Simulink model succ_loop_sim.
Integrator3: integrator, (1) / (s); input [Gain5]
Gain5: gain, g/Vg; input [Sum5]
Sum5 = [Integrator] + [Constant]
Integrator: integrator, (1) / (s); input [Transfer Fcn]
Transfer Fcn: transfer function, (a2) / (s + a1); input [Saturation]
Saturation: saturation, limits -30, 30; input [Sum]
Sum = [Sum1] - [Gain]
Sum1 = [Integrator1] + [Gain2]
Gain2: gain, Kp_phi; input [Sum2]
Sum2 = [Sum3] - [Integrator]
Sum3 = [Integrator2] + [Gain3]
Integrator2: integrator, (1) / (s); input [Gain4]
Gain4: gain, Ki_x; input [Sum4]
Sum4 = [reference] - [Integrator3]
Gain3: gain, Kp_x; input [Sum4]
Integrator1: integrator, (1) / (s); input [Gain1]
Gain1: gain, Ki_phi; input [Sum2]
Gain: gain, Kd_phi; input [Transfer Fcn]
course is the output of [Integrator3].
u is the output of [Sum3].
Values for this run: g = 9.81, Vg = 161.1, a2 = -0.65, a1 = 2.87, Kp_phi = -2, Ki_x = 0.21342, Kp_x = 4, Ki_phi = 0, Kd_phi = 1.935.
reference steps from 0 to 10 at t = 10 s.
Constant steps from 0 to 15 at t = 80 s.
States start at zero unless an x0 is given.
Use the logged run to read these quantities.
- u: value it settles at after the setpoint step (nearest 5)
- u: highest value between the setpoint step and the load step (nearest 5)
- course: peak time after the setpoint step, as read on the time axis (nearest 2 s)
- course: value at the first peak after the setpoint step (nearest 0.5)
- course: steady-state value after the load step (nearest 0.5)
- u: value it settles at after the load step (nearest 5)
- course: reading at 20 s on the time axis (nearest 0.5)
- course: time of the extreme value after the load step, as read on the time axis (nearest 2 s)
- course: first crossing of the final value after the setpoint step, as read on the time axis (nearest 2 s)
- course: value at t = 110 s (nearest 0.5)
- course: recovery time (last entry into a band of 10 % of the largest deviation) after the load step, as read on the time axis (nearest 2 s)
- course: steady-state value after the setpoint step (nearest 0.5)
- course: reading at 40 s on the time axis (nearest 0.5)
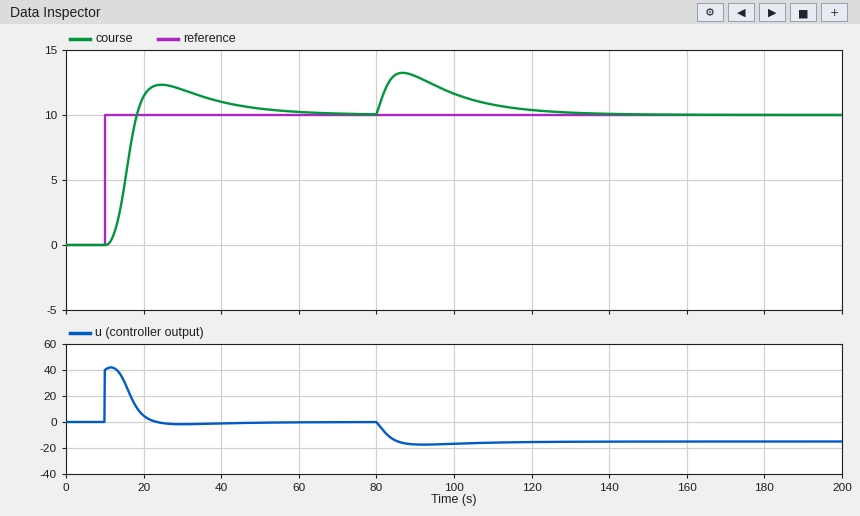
0
40
24 s
12.5
10.0
-15
11.5
86 s
18 s
11.0
122 s
10.0
11.0
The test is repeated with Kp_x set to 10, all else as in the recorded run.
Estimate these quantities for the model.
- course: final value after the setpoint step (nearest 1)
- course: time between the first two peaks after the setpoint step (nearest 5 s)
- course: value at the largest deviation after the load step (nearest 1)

10
15 s
12
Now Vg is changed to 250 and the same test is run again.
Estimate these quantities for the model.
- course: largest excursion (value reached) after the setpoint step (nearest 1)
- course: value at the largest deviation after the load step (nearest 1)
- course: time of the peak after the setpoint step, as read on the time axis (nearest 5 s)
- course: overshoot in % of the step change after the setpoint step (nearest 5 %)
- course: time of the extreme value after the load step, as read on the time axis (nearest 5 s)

13
13
30 s
25 %
90 s
